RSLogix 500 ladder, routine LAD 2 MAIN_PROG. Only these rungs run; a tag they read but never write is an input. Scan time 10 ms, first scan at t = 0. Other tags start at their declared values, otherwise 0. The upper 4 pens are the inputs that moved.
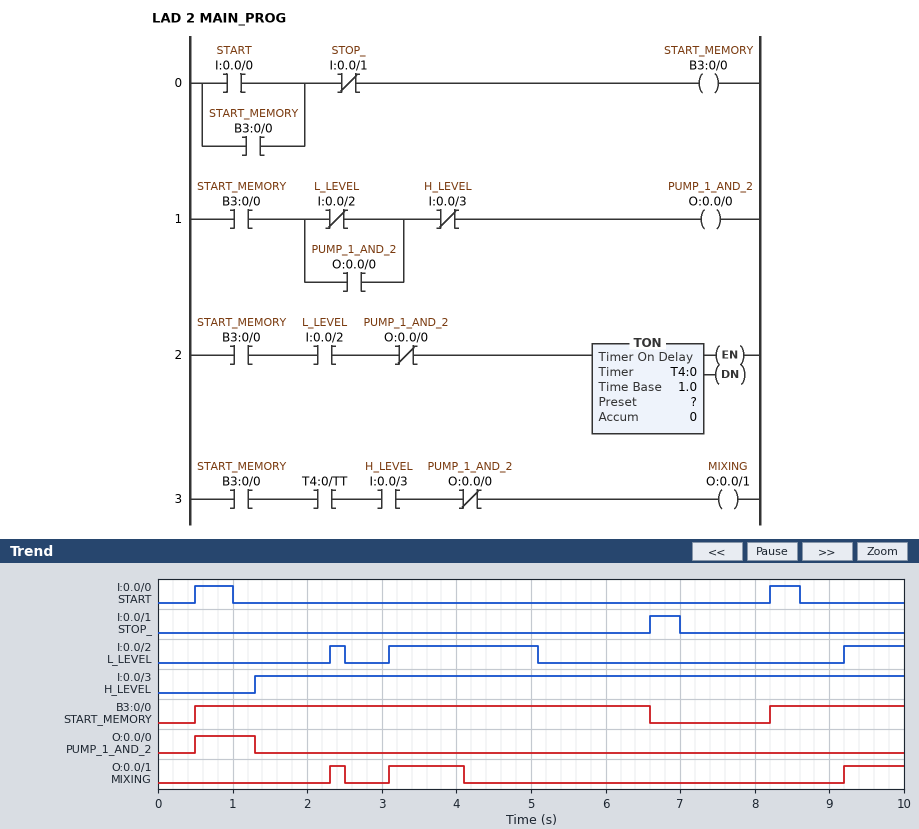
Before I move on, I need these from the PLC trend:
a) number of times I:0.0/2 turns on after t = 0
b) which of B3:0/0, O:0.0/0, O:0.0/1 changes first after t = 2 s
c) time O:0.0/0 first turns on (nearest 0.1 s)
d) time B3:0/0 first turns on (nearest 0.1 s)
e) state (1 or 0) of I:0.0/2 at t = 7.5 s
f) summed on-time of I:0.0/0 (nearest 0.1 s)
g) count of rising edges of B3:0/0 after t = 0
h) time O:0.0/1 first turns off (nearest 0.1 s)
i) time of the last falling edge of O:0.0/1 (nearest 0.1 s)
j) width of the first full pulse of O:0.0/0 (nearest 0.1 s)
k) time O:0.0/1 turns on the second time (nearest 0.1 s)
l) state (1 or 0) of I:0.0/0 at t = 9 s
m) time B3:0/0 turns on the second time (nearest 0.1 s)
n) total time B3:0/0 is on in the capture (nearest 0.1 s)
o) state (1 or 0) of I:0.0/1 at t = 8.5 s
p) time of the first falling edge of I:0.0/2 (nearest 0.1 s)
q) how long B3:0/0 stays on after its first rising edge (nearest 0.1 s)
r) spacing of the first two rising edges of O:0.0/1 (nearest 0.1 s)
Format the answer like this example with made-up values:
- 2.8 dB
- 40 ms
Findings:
- 3
- O:0.0/1
- 0.5 s
- 0.5 s
- 0
- 0.9 s
- 2
- 2.5 s
- 4.1 s
- 0.8 s
- 3.1 s
- 0
- 8.2 s
- 7.9 s
- 0
- 2.5 s
- 6.1 s
- 0.8 s
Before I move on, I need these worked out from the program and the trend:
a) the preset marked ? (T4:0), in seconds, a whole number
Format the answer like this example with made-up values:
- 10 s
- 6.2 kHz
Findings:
- 1 s
